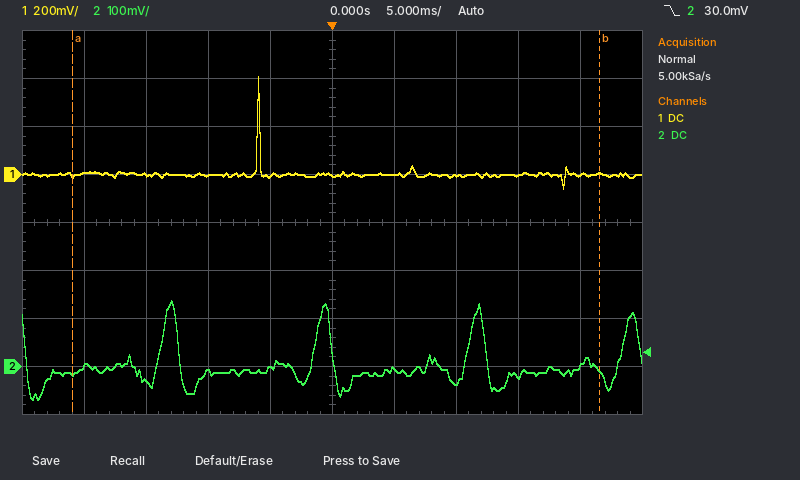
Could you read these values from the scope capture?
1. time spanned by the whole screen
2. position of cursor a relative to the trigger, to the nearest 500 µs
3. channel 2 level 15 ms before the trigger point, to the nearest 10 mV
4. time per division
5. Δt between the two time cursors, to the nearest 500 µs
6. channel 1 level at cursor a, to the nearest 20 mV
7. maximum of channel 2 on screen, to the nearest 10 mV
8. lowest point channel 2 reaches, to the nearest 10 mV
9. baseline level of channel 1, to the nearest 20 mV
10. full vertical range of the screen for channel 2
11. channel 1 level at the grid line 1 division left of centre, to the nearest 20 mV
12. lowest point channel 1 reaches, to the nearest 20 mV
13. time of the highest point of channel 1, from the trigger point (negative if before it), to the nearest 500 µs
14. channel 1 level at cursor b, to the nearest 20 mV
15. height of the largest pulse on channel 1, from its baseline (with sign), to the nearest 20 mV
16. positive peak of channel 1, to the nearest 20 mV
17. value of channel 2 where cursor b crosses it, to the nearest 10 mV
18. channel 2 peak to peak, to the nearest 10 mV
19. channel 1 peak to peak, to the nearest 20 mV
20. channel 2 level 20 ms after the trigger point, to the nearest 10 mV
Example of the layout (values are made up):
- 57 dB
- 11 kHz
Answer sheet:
- 50 ms
- -21.0 ms
- -30 mV
- 5 ms
- 42.5 ms
- 0 mV
- 140 mV
- -70 mV
- 0 mV
- 800 mV
- 0 mV
- -60 mV
- -6.0 ms
- 0 mV
- +400 mV
- 400 mV
- -10 mV
- 210 mV
- 460 mV
- 0 mV
